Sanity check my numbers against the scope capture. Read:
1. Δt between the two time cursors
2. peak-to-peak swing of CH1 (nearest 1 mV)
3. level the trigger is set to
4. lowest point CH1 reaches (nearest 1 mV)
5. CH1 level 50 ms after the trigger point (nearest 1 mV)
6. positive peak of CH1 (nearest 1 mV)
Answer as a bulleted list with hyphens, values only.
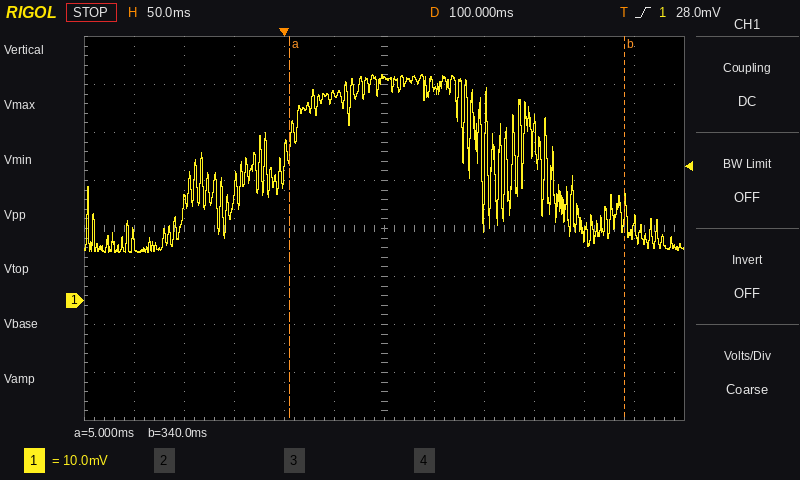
- 335 ms
- 37 mV
- 28.0 mV
- 10 mV
- 43 mV
- 47 mV
